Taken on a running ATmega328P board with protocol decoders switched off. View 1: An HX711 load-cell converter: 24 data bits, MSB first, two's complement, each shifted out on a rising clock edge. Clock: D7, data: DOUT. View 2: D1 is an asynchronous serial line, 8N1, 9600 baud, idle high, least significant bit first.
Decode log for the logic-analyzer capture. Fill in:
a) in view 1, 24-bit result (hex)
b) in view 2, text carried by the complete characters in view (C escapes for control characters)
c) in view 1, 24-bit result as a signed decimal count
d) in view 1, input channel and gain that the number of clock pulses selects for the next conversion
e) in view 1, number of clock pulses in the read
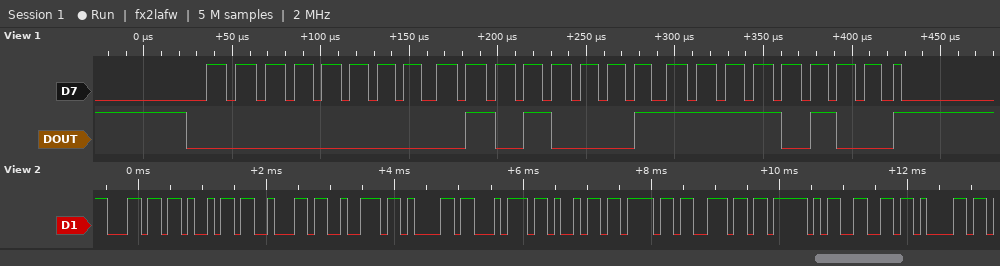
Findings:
0x0051F4
"libration_fa"
20980
channel A, gain 128
25
